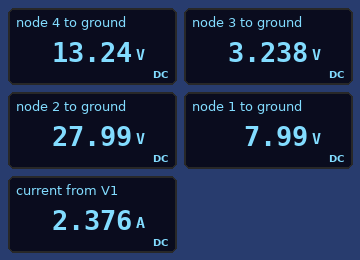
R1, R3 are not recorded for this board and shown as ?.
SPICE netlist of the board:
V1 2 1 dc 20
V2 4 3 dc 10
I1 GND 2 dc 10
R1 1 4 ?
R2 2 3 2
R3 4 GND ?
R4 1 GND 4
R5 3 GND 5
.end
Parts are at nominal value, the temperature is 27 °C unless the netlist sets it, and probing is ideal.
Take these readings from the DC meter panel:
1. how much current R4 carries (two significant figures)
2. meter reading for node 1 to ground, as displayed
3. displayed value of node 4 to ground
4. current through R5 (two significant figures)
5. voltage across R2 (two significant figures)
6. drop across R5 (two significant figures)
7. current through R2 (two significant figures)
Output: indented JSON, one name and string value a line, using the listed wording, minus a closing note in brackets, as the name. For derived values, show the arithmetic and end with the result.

{
  "how much current R4 carries": "(7.99 V) / 4 Ω = 2.0 A",
  "meter reading for node 1 to ground, as displayed": "7.99 V",
  "displayed value of node 4 to ground": "13.24 V",
  "current through R5": "(3.238 V) / 5 Ω = 650 mA",
  "voltage across R2": "27.99 V - 3.238 V = 25 V",
  "drop across R5": "3.238 V = 3.2 V",
  "current through R2": "(27.99 V - 3.238 V) / 2 Ω = 12 A"
}
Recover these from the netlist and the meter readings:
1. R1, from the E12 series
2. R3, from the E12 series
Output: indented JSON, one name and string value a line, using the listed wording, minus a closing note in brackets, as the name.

{
  "R1, from the E12 series": "1.2 Ω",
  "R3, from the E12 series": "1.8 Ω"
}
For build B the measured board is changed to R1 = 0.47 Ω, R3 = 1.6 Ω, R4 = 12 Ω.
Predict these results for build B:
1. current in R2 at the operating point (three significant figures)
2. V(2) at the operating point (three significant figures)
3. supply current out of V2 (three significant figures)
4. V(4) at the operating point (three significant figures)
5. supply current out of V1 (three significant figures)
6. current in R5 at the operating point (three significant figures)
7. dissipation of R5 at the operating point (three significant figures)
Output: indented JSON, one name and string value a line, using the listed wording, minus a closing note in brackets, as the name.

{
  "current in R2 at the operating point": "13.9 A",
  "V(2) at the operating point": "31.2 V",
  "supply current out of V2": "13.2 A",
  "V(4) at the operating point": "13.4 V",
  "supply current out of V1": "3.87 A",
  "current in R5 at the operating point": "684 mA",
  "dissipation of R5 at the operating point": "2.34 W"
}
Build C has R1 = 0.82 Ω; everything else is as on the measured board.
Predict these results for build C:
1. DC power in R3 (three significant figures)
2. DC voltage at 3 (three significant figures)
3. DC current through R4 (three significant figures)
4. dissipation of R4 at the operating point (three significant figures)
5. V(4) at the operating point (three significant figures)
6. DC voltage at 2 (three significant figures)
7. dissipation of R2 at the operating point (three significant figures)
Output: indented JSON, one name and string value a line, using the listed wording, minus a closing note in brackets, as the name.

{
  "DC power in R3": "93.5 W",
  "DC voltage at 3": "2.97 V",
  "DC current through R4": "2.20 A",
  "dissipation of R4 at the operating point": "19.3 W",
  "V(4) at the operating point": "13.0 V",
  "DC voltage at 2": "28.8 V",
  "dissipation of R2 at the operating point": "333 W"
}
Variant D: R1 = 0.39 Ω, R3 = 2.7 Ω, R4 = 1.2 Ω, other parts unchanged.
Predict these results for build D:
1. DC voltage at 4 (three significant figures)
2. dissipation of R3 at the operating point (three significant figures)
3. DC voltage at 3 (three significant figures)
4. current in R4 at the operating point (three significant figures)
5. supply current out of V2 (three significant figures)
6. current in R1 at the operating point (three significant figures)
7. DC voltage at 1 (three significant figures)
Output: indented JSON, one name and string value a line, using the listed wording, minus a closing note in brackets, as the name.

{
  "DC voltage at 4": "10.7 V",
  "dissipation of R3 at the operating point": "42.1 W",
  "DC voltage at 3": "664 mV",
  "current in R4 at the operating point": "5.92 A",
  "supply current out of V2": "13.1 A",
  "current in R1 at the operating point": "9.14 A",
  "DC voltage at 1": "7.10 V"
}
